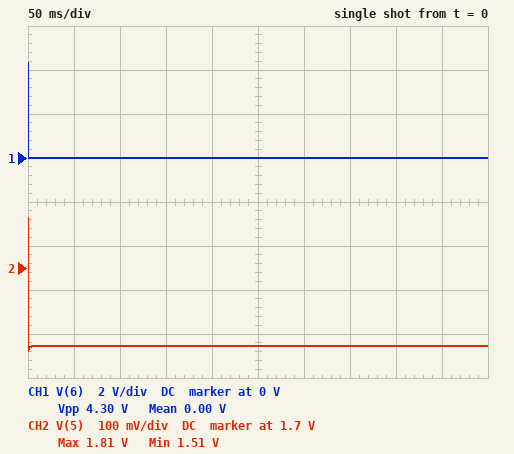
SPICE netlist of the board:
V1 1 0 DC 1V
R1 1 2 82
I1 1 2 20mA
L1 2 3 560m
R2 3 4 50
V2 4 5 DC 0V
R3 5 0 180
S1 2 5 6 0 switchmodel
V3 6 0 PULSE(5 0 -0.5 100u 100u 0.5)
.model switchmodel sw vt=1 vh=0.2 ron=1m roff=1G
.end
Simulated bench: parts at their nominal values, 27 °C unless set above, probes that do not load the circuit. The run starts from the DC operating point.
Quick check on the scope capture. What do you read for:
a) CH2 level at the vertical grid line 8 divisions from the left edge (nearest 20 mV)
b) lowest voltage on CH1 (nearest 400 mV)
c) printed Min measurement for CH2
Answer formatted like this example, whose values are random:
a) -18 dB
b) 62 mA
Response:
a) 1.52 V
b) 0 V
c) 1.51 V
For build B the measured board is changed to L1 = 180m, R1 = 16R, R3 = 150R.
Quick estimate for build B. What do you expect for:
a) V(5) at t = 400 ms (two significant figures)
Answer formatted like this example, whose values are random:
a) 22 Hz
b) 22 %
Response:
a) 920 mV
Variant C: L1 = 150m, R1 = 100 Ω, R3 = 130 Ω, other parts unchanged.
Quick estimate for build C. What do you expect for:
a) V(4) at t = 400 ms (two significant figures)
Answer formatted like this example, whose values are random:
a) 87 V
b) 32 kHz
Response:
a) 1.4 V
